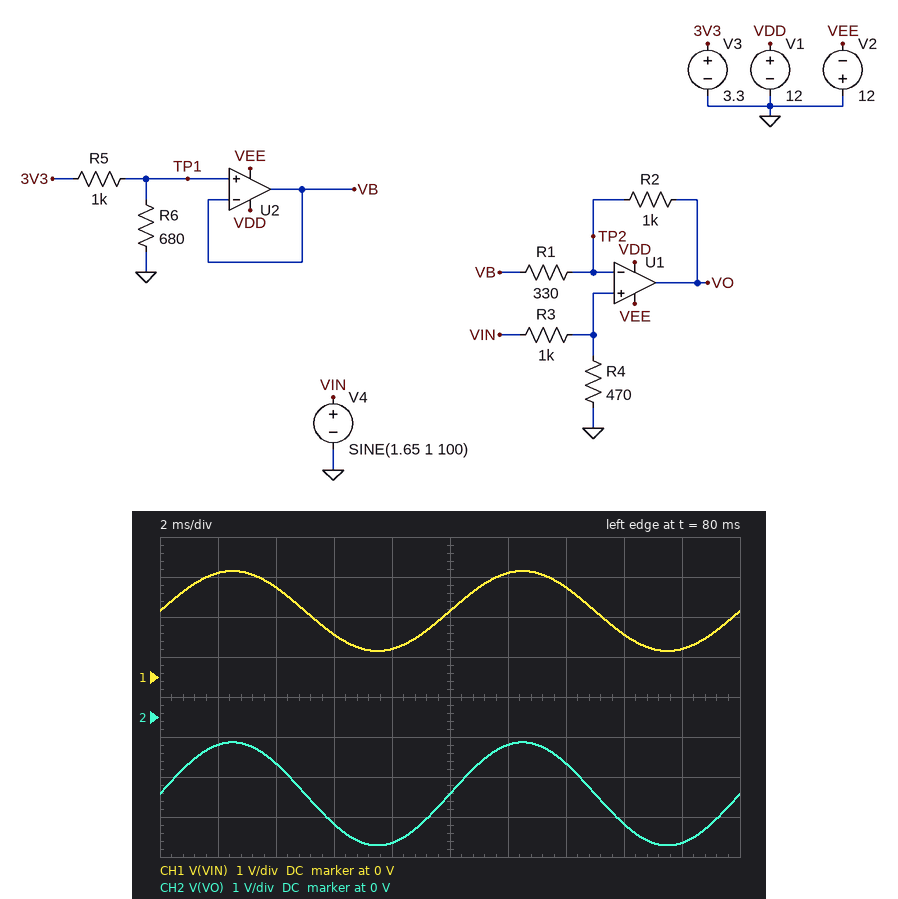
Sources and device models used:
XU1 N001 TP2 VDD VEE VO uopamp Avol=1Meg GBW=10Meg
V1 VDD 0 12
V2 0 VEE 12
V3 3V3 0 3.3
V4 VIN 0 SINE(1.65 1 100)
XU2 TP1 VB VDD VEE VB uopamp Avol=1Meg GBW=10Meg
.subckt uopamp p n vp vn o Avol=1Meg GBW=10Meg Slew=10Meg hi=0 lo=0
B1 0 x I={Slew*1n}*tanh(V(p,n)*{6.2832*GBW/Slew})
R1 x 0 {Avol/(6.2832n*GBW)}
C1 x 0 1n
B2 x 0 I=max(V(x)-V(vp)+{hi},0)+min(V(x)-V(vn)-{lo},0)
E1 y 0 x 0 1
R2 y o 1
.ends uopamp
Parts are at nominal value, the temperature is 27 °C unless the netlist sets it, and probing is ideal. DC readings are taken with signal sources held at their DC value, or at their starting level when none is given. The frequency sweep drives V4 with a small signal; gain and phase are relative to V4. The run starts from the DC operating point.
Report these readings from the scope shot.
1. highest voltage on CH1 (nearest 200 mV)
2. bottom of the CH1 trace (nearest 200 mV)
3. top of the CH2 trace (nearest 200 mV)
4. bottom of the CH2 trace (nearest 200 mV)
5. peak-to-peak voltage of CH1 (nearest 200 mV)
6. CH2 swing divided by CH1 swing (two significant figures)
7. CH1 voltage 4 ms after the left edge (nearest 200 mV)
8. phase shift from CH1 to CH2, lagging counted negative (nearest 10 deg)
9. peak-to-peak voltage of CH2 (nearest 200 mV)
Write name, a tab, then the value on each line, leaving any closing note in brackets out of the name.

highest voltage on CH1	2.6 V
bottom of the CH1 trace	600 mV
top of the CH2 trace	-600 mV
bottom of the CH2 trace	-3.2 V
peak-to-peak voltage of CH1	2.0 V
CH2 swing divided by CH1 swing	1.3
CH1 voltage 4 ms after the left edge	2.2 V
phase shift from CH1 to CH2, lagging counted negative	0 deg
peak-to-peak voltage of CH2	2.6 V
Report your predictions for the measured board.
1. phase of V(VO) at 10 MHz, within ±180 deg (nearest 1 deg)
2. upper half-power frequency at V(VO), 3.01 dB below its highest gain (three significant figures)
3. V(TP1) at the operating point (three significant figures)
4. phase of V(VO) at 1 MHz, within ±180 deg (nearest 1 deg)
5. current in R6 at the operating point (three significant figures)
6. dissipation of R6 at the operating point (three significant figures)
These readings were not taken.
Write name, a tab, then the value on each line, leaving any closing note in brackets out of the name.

phase of V(VO) at 10 MHz, within ±180 deg	-76 deg
upper half-power frequency at V(VO), 3.01 dB below its highest gain	2.48 MHz
V(TP1) at the operating point	1.34 V
phase of V(VO) at 1 MHz, within ±180 deg	-22 deg
current in R6 at the operating point	1.96 mA
dissipation of R6 at the operating point	2.62 mW
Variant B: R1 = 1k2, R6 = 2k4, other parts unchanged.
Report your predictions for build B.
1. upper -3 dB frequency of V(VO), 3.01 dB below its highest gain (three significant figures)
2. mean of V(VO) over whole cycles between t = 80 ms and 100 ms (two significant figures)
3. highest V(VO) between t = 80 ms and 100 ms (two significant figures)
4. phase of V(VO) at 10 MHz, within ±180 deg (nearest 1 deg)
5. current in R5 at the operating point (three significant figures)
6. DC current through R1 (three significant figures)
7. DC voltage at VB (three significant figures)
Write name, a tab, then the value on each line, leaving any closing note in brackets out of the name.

upper -3 dB frequency of V(VO), 3.01 dB below its highest gain	5.45 MHz
mean of V(VO) over whole cycles between t = 80 ms and 100 ms	-970 mV
highest V(VO) between t = 80 ms and 100 ms	-390 mV
phase of V(VO) at 10 MHz, within ±180 deg	-61 deg
current in R5 at the operating point	971 µA
DC current through R1	1.50 mA
DC voltage at VB	2.33 V
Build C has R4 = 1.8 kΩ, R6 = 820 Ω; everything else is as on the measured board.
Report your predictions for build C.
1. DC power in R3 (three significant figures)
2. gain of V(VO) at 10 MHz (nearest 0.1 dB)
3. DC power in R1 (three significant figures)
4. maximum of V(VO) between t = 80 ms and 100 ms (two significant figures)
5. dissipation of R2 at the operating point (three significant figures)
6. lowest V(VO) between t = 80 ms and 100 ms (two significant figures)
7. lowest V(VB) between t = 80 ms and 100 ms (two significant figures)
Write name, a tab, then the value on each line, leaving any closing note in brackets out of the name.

DC power in R3	347 µW
gain of V(VO) at 10 MHz	-4.1 dB
DC power in R1	550 µW
maximum of V(VO) between t = 80 ms and 100 ms	2.4 V
dissipation of R2 at the operating point	1.67 mW
lowest V(VO) between t = 80 ms and 100 ms	-2.8 V
lowest V(VB) between t = 80 ms and 100 ms	1.5 V
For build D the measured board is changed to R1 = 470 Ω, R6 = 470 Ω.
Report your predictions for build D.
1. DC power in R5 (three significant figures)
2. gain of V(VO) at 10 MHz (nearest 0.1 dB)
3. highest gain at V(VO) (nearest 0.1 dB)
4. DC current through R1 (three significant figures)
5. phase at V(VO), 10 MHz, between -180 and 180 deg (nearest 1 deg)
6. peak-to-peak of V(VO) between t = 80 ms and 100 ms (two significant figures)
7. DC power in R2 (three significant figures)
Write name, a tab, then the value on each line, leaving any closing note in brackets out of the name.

DC power in R5	5.04 mW
gain of V(VO) at 10 MHz	-10.3 dB
highest gain at V(VO)	0 dB
DC current through R1	1.12 mA
phase at V(VO), 10 MHz, between -180 and 180 deg	-72 deg
peak-to-peak of V(VO) between t = 80 ms and 100 ms	2.0 V
DC power in R2	1.26 mW
